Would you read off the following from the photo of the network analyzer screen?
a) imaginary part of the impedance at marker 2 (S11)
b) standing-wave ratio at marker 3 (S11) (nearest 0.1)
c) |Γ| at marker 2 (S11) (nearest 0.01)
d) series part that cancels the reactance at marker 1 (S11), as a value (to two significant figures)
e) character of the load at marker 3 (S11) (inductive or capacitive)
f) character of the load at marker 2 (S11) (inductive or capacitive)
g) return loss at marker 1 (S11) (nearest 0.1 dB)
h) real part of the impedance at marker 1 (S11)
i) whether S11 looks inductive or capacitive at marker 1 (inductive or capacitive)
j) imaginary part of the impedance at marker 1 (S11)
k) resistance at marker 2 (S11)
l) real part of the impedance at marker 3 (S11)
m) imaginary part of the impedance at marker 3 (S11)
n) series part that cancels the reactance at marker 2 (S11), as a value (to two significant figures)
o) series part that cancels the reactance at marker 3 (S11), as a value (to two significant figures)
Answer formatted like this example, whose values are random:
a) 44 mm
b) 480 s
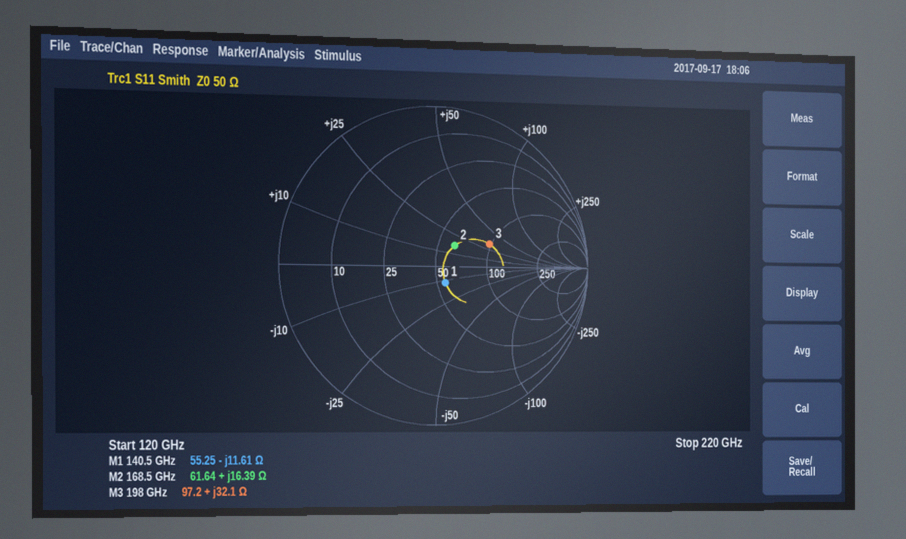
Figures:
a) +16.39 Ω
b) 2.2
c) 0.18
d) 13 pH
e) inductive
f) inductive
g) 18.4 dB
h) 55.25 Ω
i) capacitive
j) -11.61 Ω
k) 61.64 Ω
l) 97.2 Ω
m) +32.1 Ω
n) 58 fF
o) 25 fF
